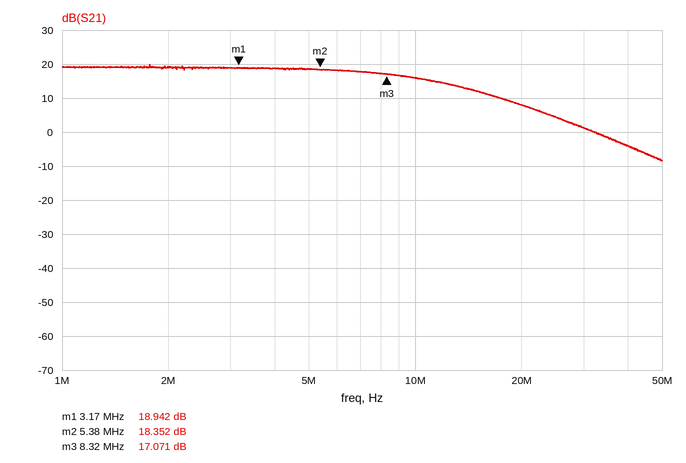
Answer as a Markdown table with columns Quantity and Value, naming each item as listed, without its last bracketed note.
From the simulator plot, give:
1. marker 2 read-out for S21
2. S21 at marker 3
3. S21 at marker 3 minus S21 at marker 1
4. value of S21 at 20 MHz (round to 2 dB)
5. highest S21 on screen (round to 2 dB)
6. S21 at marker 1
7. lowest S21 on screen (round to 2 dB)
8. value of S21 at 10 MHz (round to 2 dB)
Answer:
| Quantity | Value |
|---|---|
| marker 2 read-out for S21 | 18.352 dB |
| S21 at marker 3 | 17.071 dB |
| S21 at marker 3 minus S21 at marker 1 | -1.871 dB |
| value of S21 at 20 MHz | 8 dB |
| highest S21 on screen | 20 dB |
| S21 at marker 1 | 18.942 dB |
| lowest S21 on screen | -8 dB |
| value of S21 at 10 MHz | 16 dB |
